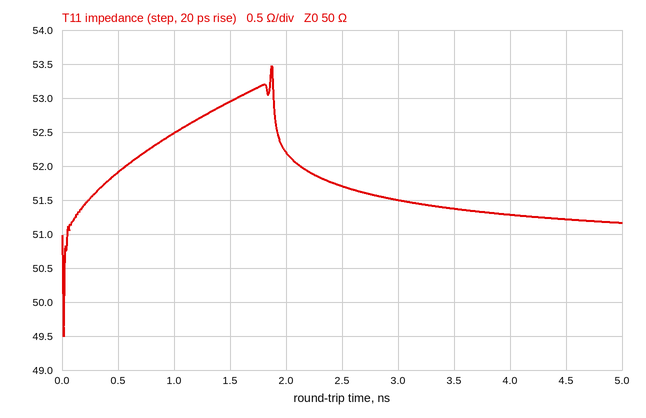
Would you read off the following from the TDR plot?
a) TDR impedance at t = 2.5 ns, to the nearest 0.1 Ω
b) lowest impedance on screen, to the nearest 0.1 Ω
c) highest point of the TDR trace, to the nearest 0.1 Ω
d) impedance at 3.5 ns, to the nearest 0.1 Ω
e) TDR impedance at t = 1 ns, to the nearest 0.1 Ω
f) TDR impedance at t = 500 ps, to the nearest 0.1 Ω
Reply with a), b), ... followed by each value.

a) 51.7 Ω
b) 49.5 Ω
c) 53.5 Ω
d) 51.4 Ω
e) 52.5 Ω
f) 51.9 Ω
